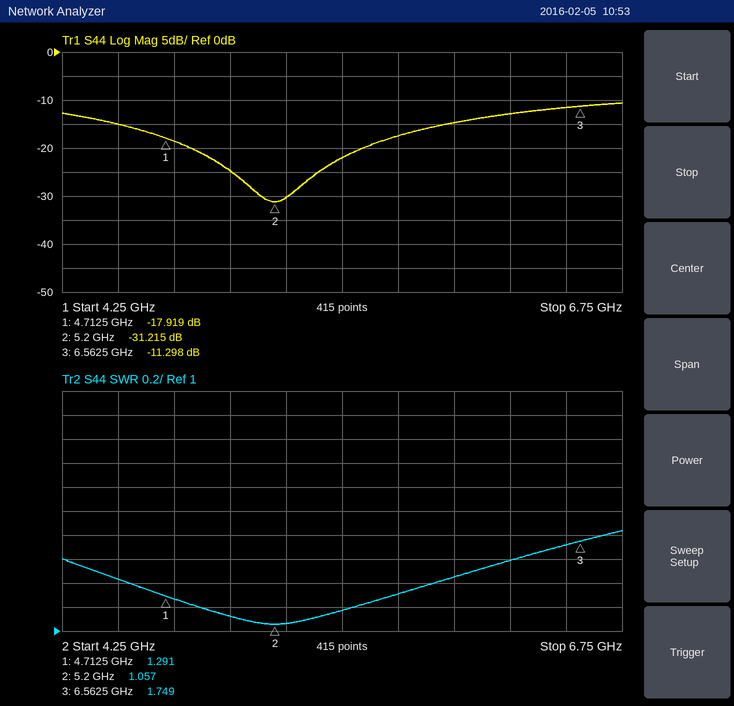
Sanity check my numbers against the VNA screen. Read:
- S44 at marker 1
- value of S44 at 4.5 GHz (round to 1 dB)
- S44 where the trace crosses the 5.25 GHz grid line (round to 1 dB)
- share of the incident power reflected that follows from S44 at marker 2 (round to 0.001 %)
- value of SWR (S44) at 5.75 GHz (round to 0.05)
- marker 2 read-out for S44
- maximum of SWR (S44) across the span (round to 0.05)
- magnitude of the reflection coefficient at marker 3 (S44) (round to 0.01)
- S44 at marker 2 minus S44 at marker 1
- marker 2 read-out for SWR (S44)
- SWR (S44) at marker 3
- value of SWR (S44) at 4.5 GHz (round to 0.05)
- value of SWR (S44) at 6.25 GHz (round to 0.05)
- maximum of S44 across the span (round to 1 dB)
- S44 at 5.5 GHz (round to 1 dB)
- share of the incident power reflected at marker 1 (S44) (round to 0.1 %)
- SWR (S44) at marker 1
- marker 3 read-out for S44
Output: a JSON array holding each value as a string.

["-17.919 dB", "-15 dB", "-30 dB", "0.076 %", "1.30", "-31.215 dB", "1.85", "0.27", "-13.296 dB", "1.057", "1.749", "1.45", "1.60", "-11 dB", "-22 dB", "1.6 %", "1.291", "-11.298 dB"]
